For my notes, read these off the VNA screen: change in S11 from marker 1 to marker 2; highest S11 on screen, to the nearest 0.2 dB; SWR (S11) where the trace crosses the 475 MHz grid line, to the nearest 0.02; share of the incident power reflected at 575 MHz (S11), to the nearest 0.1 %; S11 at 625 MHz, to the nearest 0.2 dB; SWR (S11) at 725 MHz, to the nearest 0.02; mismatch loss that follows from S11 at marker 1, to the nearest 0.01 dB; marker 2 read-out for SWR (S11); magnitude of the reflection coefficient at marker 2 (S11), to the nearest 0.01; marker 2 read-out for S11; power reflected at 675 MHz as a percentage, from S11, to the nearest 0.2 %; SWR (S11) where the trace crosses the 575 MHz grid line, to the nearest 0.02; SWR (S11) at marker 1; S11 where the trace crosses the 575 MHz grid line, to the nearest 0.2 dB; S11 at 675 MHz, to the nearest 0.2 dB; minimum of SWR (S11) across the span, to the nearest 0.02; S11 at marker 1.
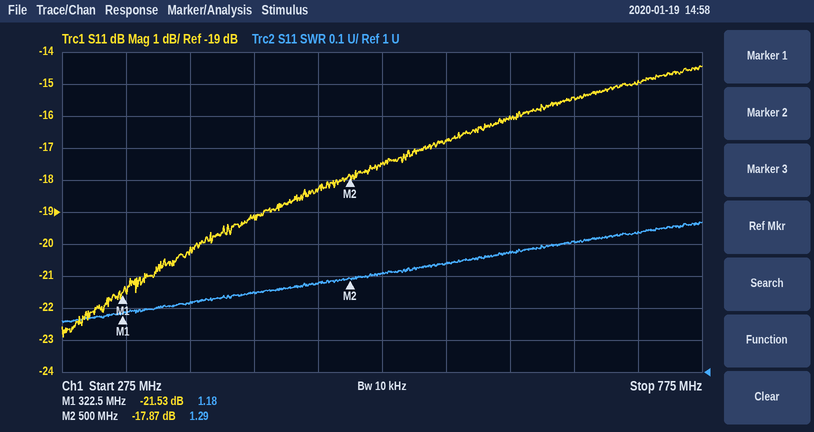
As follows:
3.66 dB
-14.4 dB
1.28
2.1 %
-16.0 dB
1.44
0.03 dB
1.29
0.13
-17.87 dB
2.8 %
1.34
1.18
-16.8 dB
-15.4 dB
1.16
-21.53 dB
